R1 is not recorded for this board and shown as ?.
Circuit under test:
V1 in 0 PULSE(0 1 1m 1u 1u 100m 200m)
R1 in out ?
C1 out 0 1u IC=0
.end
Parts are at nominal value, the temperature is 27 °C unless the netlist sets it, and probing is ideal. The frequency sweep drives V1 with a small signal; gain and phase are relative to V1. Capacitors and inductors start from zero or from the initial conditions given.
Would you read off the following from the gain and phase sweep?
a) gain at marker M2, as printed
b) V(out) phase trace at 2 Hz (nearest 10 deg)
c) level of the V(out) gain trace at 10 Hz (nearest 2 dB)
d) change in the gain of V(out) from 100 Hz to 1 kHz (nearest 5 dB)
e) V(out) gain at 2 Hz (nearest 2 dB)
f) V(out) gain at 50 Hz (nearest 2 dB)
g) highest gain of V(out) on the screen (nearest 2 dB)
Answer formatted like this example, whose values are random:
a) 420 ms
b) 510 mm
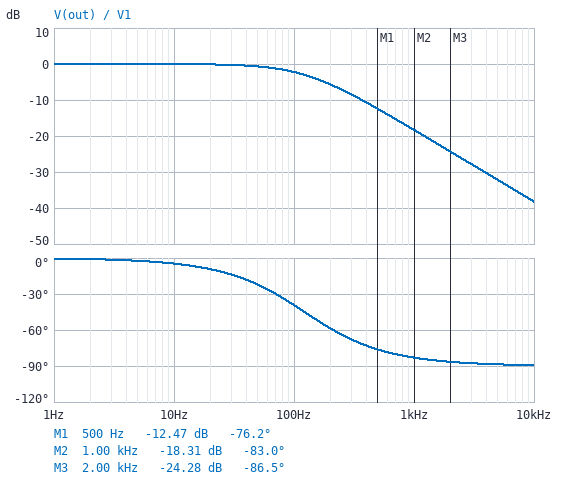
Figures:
a) -18.31 dB
b) 0 deg
c) 0 dB
d) -15 dB
e) 0 dB
f) 0 dB
g) 0 dB
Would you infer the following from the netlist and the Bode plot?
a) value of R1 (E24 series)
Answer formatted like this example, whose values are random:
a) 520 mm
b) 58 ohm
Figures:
a) 1.3 kΩ
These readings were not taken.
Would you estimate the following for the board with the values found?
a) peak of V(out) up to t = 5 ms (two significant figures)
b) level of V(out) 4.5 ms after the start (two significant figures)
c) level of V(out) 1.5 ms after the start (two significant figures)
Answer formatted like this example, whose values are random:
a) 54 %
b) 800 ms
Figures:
a) 950 mV
b) 930 mV
c) 320 mV
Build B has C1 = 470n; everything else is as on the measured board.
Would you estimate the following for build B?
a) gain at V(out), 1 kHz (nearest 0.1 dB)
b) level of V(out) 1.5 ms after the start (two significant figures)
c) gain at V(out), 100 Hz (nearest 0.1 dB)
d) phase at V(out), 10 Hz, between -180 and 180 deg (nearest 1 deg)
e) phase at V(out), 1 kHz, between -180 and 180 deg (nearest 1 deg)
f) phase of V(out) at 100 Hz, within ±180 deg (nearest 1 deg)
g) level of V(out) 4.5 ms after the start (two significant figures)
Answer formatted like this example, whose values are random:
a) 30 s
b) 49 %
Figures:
a) -12.0 dB
b) 560 mV
c) -0.6 dB
d) -2 deg
e) -75 deg
f) -21 deg
g) 1.0 V
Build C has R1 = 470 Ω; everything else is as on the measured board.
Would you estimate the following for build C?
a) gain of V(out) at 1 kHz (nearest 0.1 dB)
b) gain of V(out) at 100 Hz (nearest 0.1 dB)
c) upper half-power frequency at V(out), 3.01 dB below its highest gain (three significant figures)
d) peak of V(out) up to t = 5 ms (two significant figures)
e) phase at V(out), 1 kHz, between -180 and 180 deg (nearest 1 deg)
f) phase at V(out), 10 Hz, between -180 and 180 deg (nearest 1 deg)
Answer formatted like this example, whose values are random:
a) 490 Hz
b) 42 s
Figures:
a) -9.9 dB
b) -0.4 dB
c) 339 Hz
d) 1.0 V
e) -71 deg
f) -2 deg
